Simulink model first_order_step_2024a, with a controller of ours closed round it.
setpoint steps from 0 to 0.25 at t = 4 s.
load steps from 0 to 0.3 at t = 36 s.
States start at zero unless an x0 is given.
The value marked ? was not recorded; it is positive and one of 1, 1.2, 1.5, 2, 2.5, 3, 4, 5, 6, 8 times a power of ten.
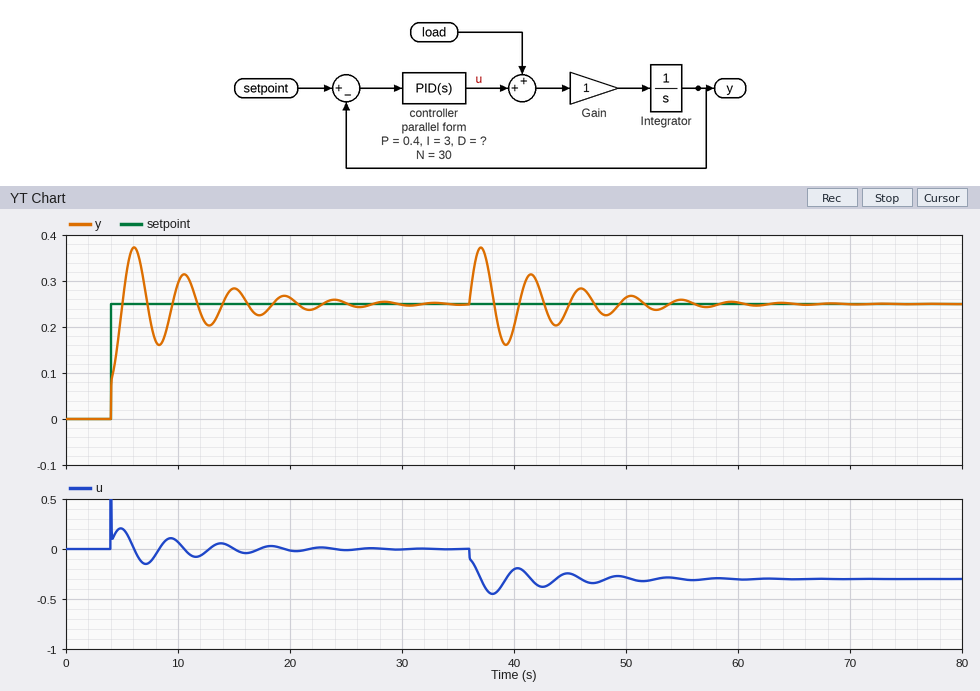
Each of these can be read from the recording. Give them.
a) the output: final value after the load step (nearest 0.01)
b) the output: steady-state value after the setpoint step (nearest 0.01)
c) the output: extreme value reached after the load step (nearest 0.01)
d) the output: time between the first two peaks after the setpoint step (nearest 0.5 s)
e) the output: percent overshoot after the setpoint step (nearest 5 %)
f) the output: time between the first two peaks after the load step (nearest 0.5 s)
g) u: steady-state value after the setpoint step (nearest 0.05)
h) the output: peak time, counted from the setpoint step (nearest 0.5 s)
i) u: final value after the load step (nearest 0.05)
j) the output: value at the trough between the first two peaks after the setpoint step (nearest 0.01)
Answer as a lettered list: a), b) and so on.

a) 0.25
b) 0.25
c) 0.37
d) 4.5 s
e) 50 %
f) 4.5 s
g) 0.00
h) 2.0 s
i) -0.30
j) 0.16
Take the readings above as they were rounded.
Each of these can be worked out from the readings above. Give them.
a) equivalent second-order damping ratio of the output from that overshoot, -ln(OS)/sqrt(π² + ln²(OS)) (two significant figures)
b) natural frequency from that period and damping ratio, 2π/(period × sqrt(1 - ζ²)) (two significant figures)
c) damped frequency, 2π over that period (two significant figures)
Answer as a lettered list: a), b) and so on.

a) 0.22
b) 1.4 rad/s
c) 1.4 rad/s
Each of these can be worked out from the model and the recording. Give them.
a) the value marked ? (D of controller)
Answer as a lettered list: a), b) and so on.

a) 0.5
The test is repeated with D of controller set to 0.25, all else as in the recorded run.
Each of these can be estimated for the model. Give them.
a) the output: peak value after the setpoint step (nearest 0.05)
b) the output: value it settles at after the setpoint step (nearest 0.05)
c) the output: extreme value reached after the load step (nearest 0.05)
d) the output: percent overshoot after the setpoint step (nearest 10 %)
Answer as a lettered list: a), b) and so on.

a) 0.40
b) 0.25
c) 0.40
d) 60 %
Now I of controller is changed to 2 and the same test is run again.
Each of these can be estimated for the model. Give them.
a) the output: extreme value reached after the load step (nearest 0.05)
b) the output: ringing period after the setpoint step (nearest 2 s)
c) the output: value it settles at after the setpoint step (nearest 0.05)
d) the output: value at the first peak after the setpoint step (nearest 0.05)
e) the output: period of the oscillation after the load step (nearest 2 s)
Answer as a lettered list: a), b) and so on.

a) 0.40
b) 6 s
c) 0.25
d) 0.35
e) 6 s
